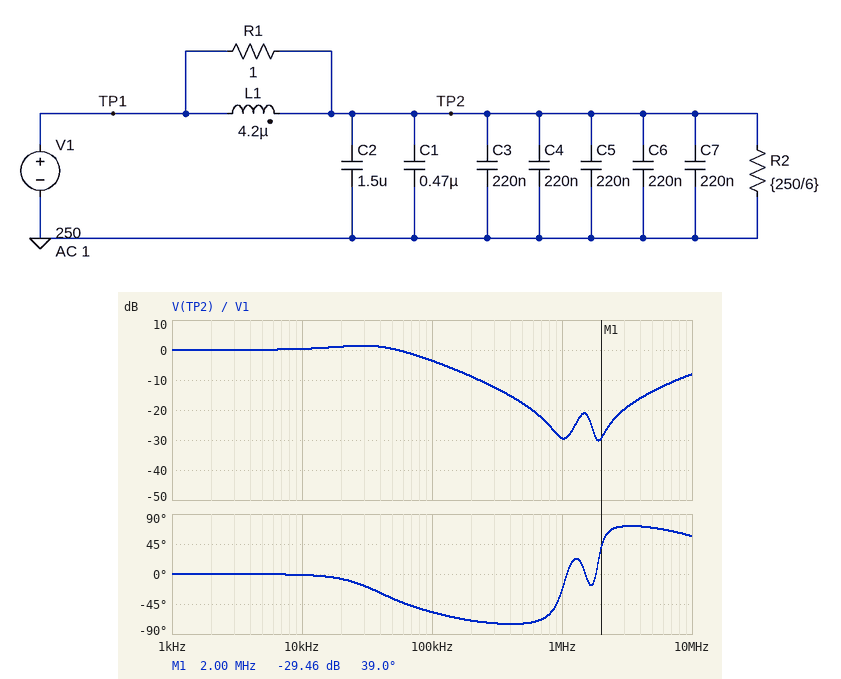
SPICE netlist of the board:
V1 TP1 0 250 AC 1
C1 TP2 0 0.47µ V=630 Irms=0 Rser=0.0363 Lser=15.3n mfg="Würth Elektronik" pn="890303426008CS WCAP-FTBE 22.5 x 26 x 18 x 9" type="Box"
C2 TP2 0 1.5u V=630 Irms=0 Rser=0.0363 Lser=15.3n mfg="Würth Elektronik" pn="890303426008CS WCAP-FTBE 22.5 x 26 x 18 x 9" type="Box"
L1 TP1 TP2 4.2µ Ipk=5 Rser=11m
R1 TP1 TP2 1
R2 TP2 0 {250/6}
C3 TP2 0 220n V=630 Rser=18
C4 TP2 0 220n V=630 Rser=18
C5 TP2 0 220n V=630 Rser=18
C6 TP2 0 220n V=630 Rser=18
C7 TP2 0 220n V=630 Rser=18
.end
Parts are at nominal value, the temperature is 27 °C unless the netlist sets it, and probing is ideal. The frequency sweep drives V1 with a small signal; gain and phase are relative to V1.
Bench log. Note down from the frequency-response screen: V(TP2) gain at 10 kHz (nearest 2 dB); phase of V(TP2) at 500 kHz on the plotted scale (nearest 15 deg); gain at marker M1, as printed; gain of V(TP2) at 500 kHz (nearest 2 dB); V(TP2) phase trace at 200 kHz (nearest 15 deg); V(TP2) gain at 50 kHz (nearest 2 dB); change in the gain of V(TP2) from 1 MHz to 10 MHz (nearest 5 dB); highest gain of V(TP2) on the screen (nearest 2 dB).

0 dB
-75 deg
-29.46 dB
-18 dB
-75 deg
0 dB
20 dB
2 dB
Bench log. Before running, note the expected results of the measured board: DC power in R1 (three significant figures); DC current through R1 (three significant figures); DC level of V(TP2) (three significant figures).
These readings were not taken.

4.26 mW
65.3 mA
250 V
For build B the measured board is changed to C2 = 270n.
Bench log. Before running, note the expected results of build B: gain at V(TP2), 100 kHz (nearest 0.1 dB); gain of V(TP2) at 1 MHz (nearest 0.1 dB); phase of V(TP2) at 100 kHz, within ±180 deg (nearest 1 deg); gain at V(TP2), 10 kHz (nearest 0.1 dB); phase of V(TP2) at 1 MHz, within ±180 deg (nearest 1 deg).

-1.6 dB
-16.1 dB
-29 deg
0.2 dB
-73 deg
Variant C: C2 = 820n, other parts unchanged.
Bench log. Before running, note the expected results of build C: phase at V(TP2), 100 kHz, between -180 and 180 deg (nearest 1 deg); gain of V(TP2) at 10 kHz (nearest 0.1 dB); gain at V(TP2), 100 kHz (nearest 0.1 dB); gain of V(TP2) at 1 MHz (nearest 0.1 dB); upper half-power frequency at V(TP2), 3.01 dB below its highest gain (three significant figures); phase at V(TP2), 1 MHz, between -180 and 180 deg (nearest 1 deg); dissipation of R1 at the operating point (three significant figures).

-43 deg
0.3 dB
-2.2 dB
-22.9 dB
95.1 kHz
-70 deg
4.26 mW
